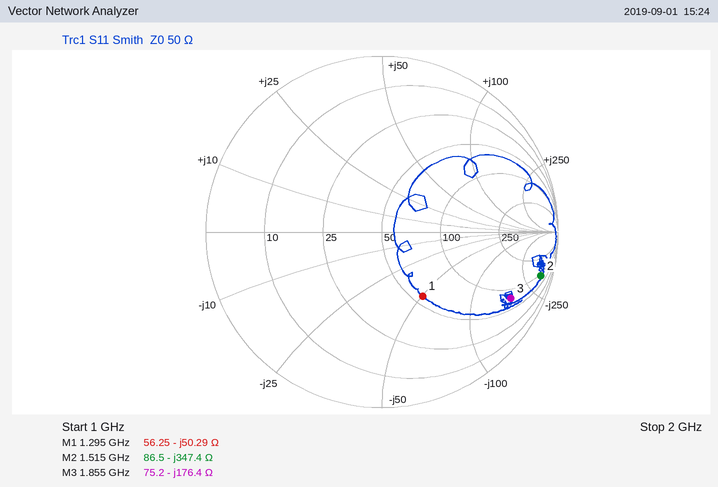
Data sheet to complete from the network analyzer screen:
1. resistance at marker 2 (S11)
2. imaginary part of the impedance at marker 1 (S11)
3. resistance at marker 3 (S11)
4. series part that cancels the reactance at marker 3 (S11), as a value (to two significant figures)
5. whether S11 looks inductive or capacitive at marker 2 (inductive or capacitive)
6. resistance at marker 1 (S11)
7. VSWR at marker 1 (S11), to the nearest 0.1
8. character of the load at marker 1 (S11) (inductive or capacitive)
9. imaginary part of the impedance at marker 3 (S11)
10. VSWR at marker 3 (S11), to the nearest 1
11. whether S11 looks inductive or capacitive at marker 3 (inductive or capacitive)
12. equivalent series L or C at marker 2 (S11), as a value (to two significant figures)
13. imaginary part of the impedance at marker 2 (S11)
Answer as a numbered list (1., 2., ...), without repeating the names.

1. 86.5 Ω
2. -50.29 Ω
3. 75.2 Ω
4. 15 nH
5. capacitive
6. 56.25 Ω
7. 2.5
8. capacitive
9. -176.4 Ω
10. 10
11. capacitive
12. 300 fF
13. -347.4 Ω
